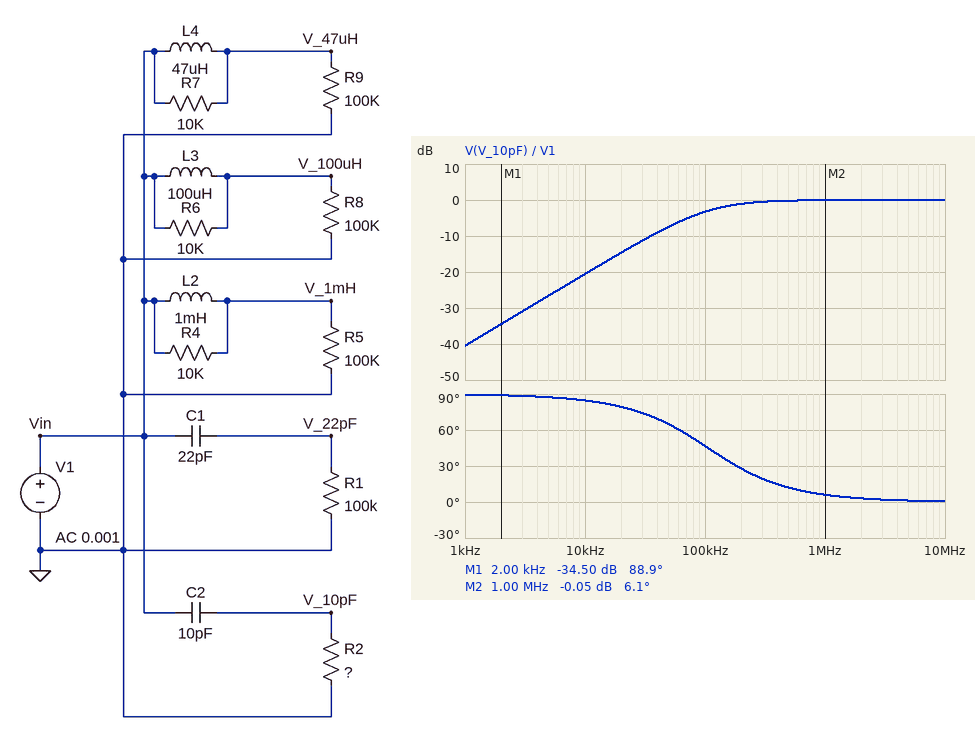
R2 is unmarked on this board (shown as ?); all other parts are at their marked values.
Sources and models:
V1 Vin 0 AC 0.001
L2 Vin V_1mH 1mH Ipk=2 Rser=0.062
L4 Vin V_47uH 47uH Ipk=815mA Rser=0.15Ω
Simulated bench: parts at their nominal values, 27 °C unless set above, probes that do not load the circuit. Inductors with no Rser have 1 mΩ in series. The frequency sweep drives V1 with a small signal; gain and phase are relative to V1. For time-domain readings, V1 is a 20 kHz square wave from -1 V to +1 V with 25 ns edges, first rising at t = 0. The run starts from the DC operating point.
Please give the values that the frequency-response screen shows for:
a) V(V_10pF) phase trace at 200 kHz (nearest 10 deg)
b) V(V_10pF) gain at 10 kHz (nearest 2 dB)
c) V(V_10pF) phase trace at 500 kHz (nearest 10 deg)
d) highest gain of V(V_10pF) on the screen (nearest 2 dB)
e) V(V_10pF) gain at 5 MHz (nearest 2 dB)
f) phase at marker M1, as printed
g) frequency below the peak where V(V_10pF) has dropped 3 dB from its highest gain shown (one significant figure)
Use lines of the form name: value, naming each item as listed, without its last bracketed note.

V(V_10pF) phase trace at 200 kHz: 30 deg
V(V_10pF) gain at 10 kHz: -20 dB
V(V_10pF) phase trace at 500 kHz: 10 deg
highest gain of V(V_10pF) on the screen: 0 dB
V(V_10pF) gain at 5 MHz: 0 dB
phase at marker M1, as printed: 88.9 deg
frequency below the peak where V(V_10pF) has dropped 3 dB from its highest gain shown: 100 kHz
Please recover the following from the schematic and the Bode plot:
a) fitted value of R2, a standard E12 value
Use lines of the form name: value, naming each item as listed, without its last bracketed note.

fitted value of R2, a standard E12 value: 150 kΩ
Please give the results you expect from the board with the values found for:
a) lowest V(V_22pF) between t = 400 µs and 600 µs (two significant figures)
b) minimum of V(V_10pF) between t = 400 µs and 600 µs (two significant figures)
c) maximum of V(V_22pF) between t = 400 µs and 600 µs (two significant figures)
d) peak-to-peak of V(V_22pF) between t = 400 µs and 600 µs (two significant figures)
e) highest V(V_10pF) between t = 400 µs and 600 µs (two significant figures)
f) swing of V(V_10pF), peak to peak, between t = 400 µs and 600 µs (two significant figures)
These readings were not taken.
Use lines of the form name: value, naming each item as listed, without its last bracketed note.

lowest V(V_22pF) between t = 400 µs and 600 µs: -2.0 V
minimum of V(V_10pF) between t = 400 µs and 600 µs: -2.0 V
maximum of V(V_22pF) between t = 400 µs and 600 µs: 2.0 V
peak-to-peak of V(V_22pF) between t = 400 µs and 600 µs: 4.0 V
highest V(V_10pF) between t = 400 µs and 600 µs: 2.0 V
swing of V(V_10pF), peak to peak, between t = 400 µs and 600 µs: 4.0 V
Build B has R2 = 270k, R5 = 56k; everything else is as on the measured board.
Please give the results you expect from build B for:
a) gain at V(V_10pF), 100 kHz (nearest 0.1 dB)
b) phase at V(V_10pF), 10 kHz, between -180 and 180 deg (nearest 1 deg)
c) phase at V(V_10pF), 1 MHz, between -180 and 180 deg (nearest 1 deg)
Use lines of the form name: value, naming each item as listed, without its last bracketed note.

gain at V(V_10pF), 100 kHz: -1.3 dB
phase at V(V_10pF), 10 kHz, between -180 and 180 deg: 80 deg
phase at V(V_10pF), 1 MHz, between -180 and 180 deg: 3 deg
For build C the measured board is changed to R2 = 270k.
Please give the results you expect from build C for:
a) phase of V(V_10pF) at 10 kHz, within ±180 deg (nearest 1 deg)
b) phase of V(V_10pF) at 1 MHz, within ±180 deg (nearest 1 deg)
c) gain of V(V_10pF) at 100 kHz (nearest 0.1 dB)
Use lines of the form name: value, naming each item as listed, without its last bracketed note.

phase of V(V_10pF) at 10 kHz, within ±180 deg: 80 deg
phase of V(V_10pF) at 1 MHz, within ±180 deg: 3 deg
gain of V(V_10pF) at 100 kHz: -1.3 dB
